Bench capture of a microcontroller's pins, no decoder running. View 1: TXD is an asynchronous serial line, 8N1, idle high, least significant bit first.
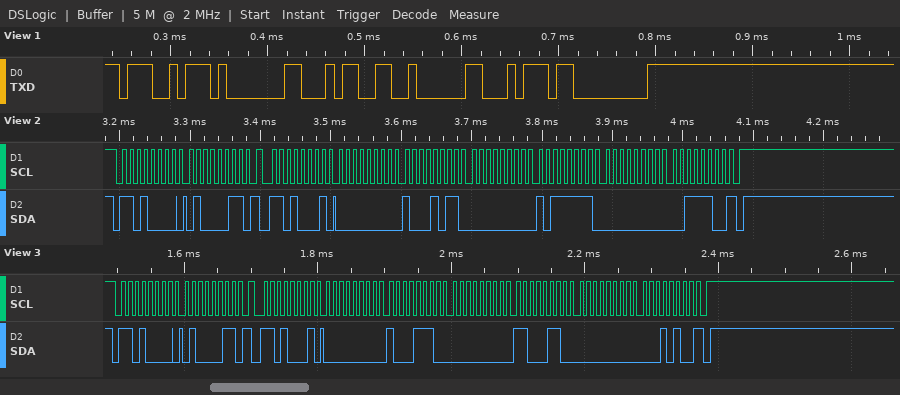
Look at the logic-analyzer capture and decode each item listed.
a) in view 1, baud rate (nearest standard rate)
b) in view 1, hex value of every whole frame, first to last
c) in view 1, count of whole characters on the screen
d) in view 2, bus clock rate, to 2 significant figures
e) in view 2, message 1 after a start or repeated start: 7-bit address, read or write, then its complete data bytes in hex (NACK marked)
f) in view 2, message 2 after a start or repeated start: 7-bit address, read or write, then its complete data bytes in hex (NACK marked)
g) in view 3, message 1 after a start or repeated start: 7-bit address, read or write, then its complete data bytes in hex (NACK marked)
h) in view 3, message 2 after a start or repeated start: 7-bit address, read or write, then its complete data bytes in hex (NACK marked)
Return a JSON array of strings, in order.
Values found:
["115200 baud", "A7 01 34 02 74 00", "6", "100 kHz", "0x68 write: 43", "0x68 read: 00 8B 00 BF 00 3C NACK", "0x68 write: 43", "0x68 read: 00 8E 00 C6 00 14 NACK"]
